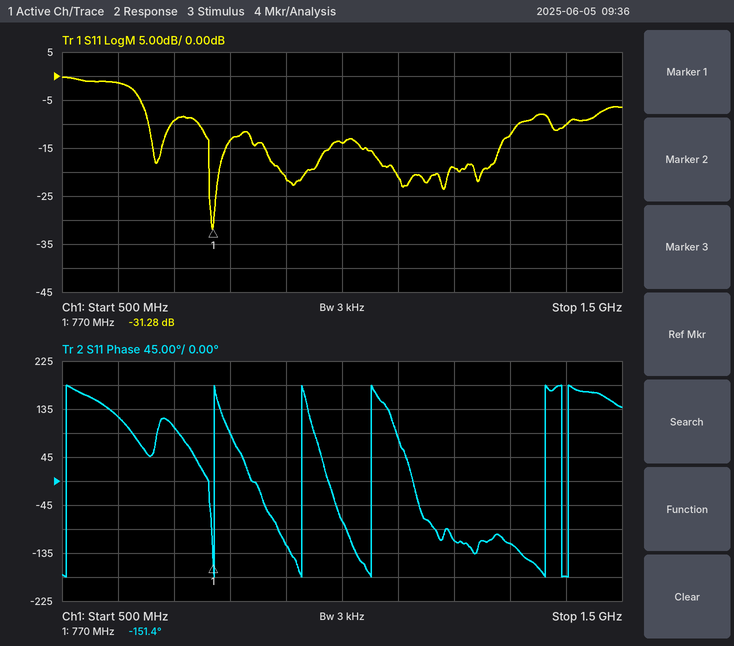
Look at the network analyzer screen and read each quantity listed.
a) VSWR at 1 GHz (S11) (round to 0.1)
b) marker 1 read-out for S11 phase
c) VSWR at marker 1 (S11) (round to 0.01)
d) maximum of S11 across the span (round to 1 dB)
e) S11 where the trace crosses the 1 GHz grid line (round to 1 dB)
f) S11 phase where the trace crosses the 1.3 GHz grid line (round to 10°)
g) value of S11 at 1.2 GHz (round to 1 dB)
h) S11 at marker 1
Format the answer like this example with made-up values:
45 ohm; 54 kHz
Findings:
1.5; -151.4°; 1.06; 0 dB; -14 dB; -120°; -19 dB; -31.28 dB
